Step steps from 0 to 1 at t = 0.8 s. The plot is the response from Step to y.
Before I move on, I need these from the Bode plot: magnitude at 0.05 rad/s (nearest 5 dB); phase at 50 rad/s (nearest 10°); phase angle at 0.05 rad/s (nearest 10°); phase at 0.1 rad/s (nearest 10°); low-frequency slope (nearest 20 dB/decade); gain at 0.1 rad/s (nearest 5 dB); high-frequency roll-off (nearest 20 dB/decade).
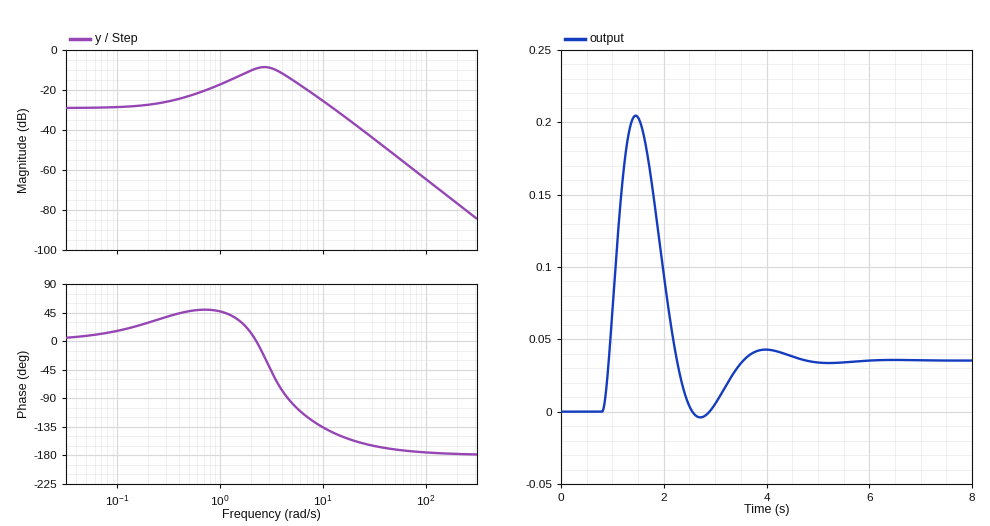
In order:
-30 dB
-170°
10°
20°
0 dB/decade
-30 dB
-40 dB/decade
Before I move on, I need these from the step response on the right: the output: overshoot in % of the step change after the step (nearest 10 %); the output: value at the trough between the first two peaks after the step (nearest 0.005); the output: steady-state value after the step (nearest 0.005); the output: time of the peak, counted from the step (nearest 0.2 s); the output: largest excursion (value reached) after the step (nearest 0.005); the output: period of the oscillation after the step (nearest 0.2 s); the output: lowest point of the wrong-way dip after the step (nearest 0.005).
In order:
480 %
-0.005
0.035
0.6 s
0.205
2.6 s
-0.005
